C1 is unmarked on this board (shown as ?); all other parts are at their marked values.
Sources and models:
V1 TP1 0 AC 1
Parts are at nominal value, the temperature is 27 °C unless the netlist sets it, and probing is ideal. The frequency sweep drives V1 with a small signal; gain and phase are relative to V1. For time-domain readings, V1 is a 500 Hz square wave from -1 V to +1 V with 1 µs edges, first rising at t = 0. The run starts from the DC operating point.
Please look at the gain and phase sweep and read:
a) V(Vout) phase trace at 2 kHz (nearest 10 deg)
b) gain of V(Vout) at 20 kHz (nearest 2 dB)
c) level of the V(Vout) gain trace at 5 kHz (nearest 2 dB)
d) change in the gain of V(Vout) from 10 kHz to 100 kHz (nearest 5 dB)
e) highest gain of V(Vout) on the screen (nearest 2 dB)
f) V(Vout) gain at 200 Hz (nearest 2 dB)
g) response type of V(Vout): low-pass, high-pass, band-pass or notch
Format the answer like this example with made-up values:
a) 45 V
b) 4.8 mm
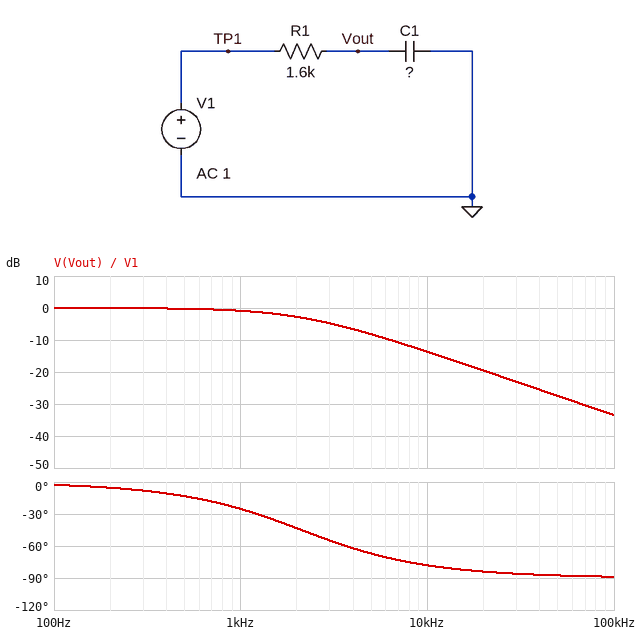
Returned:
a) -40 deg
b) -20 dB
c) -8 dB
d) -20 dB
e) 0 dB
f) 0 dB
g) low-pass
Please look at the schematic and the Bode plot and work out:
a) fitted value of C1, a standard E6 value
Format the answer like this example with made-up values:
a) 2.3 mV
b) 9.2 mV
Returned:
a) 47 nF
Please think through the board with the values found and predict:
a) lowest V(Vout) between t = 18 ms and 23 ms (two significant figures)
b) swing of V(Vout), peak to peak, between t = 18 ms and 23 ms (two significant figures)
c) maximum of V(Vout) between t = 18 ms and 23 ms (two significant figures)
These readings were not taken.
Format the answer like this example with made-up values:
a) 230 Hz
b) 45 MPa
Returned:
a) -1.0 V
b) 2.0 V
c) 1.0 V
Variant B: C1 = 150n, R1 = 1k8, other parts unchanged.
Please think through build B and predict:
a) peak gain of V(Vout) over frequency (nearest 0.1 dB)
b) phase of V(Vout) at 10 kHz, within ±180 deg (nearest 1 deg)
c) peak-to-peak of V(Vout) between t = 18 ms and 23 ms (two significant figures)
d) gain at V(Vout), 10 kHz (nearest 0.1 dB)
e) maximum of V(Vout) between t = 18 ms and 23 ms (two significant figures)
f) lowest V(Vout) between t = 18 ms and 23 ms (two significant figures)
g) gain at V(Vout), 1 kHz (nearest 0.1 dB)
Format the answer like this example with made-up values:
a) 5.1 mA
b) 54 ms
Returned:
a) 0 dB
b) -87 deg
c) 1.9 V
d) -24.6 dB
e) 950 mV
f) -950 mV
g) -5.9 dB
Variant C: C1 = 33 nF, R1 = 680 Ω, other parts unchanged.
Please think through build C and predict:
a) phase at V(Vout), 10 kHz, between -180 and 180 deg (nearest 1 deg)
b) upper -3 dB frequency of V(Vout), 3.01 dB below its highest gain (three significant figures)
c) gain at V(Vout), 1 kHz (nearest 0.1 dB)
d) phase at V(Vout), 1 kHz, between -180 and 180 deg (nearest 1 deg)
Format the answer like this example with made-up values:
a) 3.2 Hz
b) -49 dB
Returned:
a) -55 deg
b) 7.09 kHz
c) -0.1 dB
d) -8 deg
